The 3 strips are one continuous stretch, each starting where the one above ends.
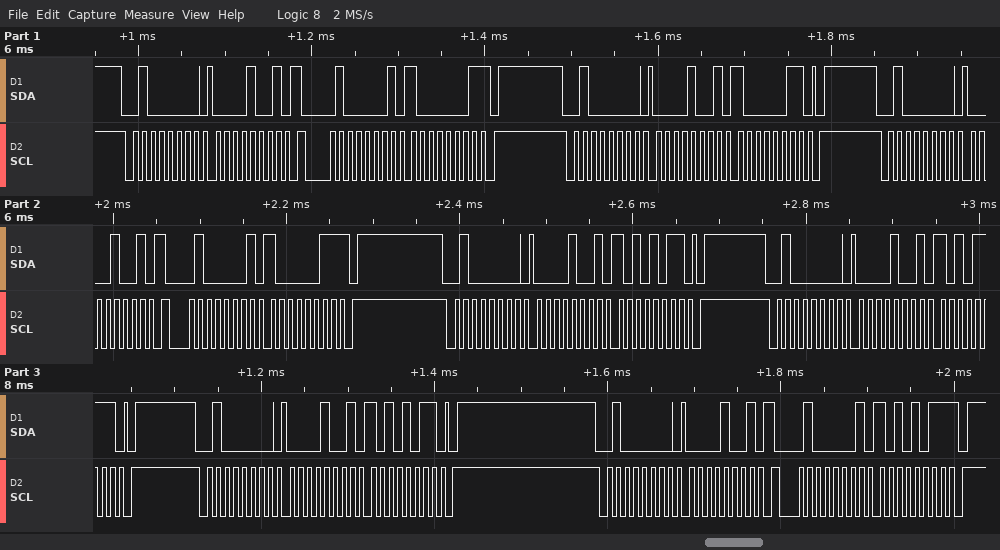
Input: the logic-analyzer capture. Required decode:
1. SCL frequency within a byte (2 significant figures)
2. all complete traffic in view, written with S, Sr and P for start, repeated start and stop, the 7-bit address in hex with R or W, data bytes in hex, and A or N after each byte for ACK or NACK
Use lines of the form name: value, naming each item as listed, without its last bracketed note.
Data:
SCL frequency within a byte: 100 kHz
all complete traffic in view, written with S, Sr and P for start, repeated start and stop, the 7-bit address in hex with R or W, data bytes in hex, and A or N after each byte for ACK or NACK: S 20W A 09 A Sr 20R A 81 N P S 20W A 09 A 83 A P S 20W A 09 A Sr 20R A 83 N P S 20W A 09 A AB A P S 20W A 09 A AF A P S 20W A 09 A AB A P S 20W A 09 A Sr 20R A AB N P
